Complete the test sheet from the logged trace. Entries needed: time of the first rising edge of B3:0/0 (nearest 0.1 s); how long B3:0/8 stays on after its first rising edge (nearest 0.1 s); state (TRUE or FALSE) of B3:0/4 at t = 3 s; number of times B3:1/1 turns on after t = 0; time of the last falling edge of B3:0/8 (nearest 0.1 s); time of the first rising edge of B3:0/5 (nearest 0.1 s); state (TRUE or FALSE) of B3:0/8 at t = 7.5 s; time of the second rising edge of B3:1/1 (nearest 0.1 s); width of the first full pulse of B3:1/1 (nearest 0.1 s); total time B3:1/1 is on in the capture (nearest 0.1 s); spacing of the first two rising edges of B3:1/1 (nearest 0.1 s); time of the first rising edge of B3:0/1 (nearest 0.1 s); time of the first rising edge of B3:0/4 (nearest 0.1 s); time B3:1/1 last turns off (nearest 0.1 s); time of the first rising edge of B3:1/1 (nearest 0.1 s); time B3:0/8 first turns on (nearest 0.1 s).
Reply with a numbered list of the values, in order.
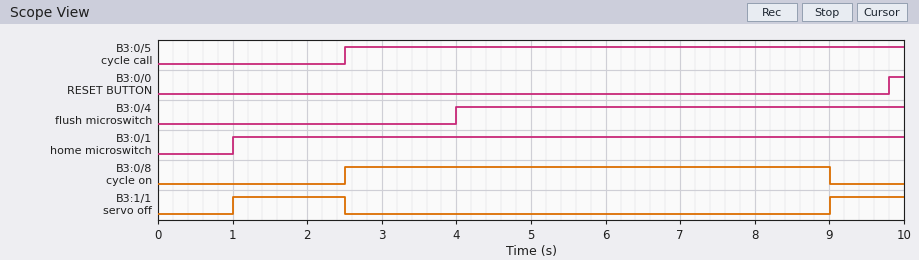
1. 9.8 s
2. 6.5 s
3. FALSE
4. 2
5. 9.0 s
6. 2.5 s
7. TRUE
8. 9.0 s
9. 1.5 s
10. 2.5 s
11. 8.0 s
12. 1.0 s
13. 4.0 s
14. 2.5 s
15. 1.0 s
16. 2.5 s
